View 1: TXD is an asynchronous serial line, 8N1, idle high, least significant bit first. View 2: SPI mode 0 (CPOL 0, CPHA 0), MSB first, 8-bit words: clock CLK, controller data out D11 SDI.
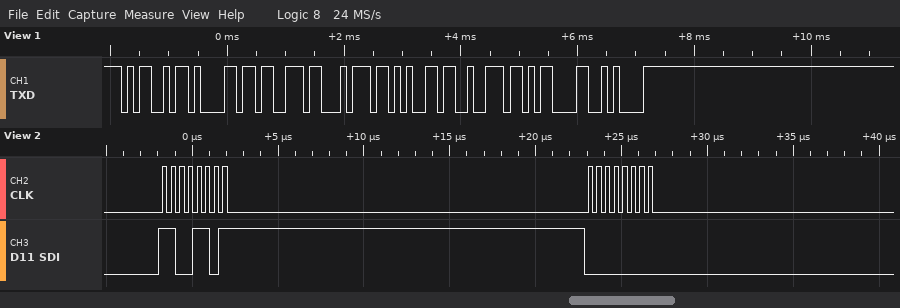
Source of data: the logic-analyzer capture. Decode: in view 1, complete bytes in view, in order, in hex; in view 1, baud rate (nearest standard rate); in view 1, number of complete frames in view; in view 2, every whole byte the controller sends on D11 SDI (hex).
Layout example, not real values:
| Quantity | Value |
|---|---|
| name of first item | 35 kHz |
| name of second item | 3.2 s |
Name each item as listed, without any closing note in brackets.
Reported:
| Quantity | Value |
|---|---|
| in view 1, complete bytes in view, in order, in hex | 4D 61 73 74 65 72 0D 0A |
| in view 1, baud rate | 9600 baud |
| in view 1, number of complete frames in view | 8 |
| in view 2, every whole byte the controller sends on D11 SDI | 0xCD 0x00 |
